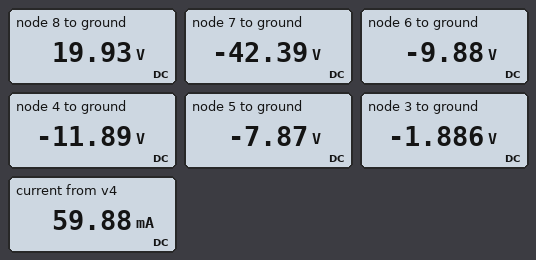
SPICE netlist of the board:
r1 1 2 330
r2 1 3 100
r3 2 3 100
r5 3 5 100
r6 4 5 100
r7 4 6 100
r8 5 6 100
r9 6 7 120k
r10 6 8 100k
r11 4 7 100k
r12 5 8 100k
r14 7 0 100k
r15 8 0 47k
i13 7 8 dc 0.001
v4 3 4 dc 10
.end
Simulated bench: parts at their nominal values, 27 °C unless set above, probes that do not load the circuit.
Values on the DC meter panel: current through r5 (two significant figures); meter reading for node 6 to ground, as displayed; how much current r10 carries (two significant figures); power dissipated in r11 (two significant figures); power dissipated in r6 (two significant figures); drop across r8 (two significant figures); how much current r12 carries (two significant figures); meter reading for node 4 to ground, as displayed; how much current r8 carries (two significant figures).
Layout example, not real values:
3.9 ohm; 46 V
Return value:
60 mA; -9.88 V; 300 µA; 9.3 mW; 160 mW; 2.0 V; 280 µA; -11.89 V; 20 mA
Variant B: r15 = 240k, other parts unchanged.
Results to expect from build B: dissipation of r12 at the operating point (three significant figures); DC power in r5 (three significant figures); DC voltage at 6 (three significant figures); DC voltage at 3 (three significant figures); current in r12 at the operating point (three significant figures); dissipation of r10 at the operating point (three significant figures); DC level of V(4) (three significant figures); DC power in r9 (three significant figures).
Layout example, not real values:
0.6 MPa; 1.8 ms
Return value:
13.7 mW; 358 mW; 18.6 V; 26.6 V; 370 µA; 15.2 mW; 16.6 V; 15.1 mW
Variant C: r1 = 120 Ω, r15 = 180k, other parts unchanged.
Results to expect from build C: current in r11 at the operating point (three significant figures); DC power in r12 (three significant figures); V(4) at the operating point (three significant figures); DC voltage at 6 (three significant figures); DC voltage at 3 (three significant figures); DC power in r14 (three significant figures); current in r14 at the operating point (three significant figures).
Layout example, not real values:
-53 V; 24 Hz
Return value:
385 µA; 12.3 mW; 10.8 V; 12.8 V; 20.8 V; 7.69 mW; 277 µA
